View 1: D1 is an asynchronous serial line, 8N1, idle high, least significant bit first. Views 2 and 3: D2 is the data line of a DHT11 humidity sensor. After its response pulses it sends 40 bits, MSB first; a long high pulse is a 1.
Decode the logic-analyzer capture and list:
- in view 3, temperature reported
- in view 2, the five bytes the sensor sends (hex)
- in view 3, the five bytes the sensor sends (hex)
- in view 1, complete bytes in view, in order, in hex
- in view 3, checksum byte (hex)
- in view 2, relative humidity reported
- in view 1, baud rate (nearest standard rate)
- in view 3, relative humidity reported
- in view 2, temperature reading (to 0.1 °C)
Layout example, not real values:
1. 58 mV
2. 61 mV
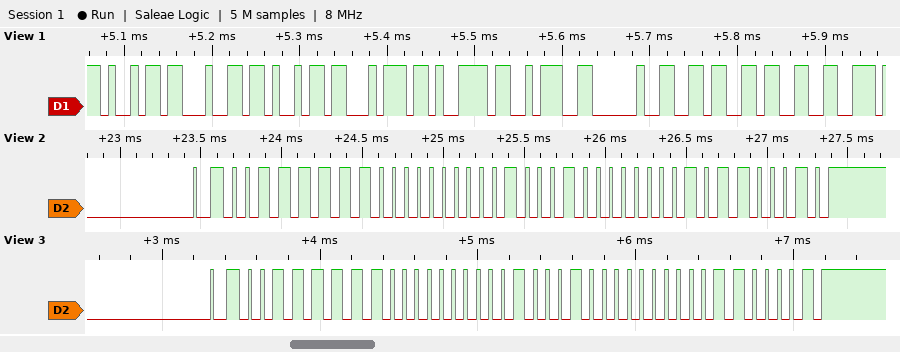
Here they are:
1. 34.0 °C
2. 3F 00 22 01 62
3. 3F 00 22 00 61
4. 69 64 69 74 79 3A 20 36 33
5. 0x61
6. 63 %
7. 115200 baud
8. 63 %
9. 34.1 °C
